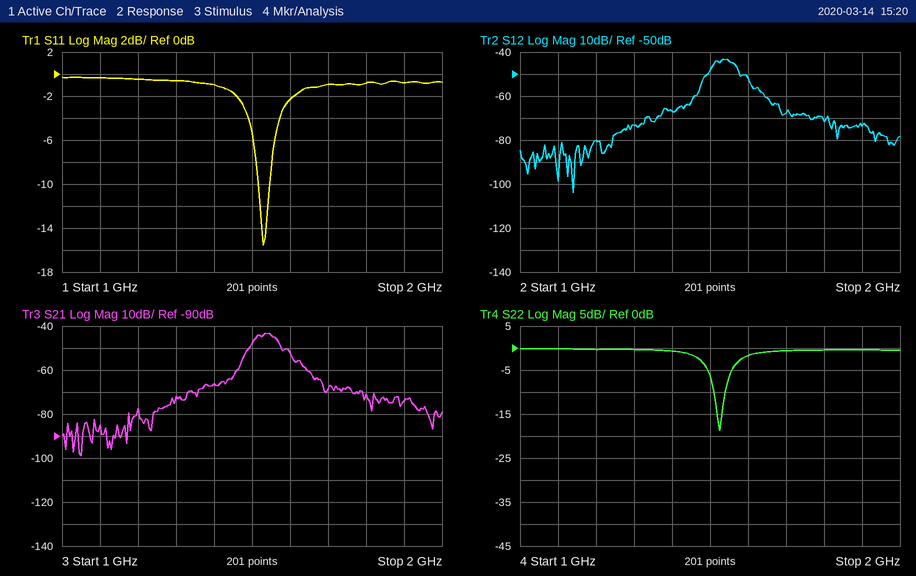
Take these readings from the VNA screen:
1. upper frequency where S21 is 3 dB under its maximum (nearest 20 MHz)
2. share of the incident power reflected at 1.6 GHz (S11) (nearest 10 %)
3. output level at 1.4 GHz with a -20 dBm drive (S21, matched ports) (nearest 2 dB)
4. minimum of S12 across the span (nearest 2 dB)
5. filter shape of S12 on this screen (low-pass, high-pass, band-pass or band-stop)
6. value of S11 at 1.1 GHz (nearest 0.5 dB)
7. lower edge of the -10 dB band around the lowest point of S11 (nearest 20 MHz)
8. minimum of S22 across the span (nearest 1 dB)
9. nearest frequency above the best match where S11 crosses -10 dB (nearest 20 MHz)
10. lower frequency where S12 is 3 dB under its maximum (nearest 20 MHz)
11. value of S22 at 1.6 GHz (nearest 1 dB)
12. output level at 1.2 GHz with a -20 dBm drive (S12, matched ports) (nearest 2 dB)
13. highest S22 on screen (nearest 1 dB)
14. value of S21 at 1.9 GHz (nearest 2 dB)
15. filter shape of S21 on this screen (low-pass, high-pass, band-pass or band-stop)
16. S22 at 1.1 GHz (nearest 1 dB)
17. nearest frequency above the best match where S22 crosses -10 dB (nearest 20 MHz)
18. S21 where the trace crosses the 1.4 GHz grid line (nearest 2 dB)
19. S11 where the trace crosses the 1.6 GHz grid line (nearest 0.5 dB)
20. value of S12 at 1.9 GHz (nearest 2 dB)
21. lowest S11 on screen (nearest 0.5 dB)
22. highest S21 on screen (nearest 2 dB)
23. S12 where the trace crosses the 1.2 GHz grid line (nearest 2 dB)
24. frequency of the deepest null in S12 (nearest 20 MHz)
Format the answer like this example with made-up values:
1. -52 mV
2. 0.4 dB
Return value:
1. 1.56 GHz
2. 60 %
3. -86 dBm
4. -104 dB
5. band-pass
6. -0.5 dB
7. 1.52 GHz
8. -19 dB
9. 1.54 GHz
10. 1.50 GHz
11. -2 dB
12. -100 dBm
13. 0 dB
14. -74 dB
15. band-pass
16. 0 dB
17. 1.54 GHz
18. -66 dB
19. -2.5 dB
20. -74 dB
21. -15.5 dB
22. -44 dB
23. -80 dB
24. 1.14 GHz
